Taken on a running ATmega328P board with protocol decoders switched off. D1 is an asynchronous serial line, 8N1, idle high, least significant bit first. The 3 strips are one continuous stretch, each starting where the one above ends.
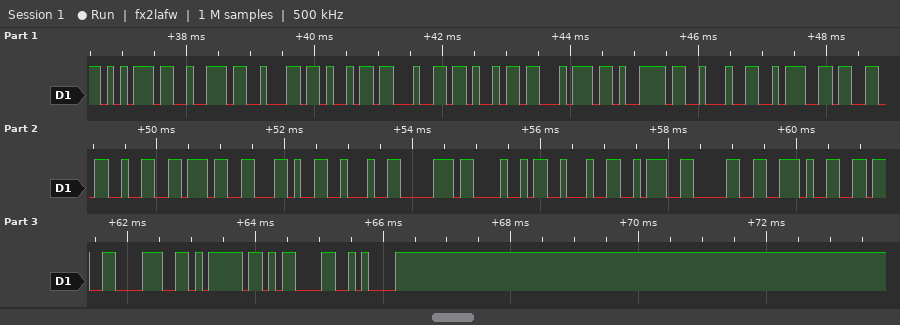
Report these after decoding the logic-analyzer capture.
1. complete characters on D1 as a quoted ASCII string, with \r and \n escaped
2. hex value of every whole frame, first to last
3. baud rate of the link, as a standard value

"urbidity\":327,\"pH\":0.68}\r\n"
75 72 62 69 64 69 74 79 22 3A 33 32 37 2C 22 70 48 22 3A 30 2E 36 38 7D 0D 0A
9600 baud
